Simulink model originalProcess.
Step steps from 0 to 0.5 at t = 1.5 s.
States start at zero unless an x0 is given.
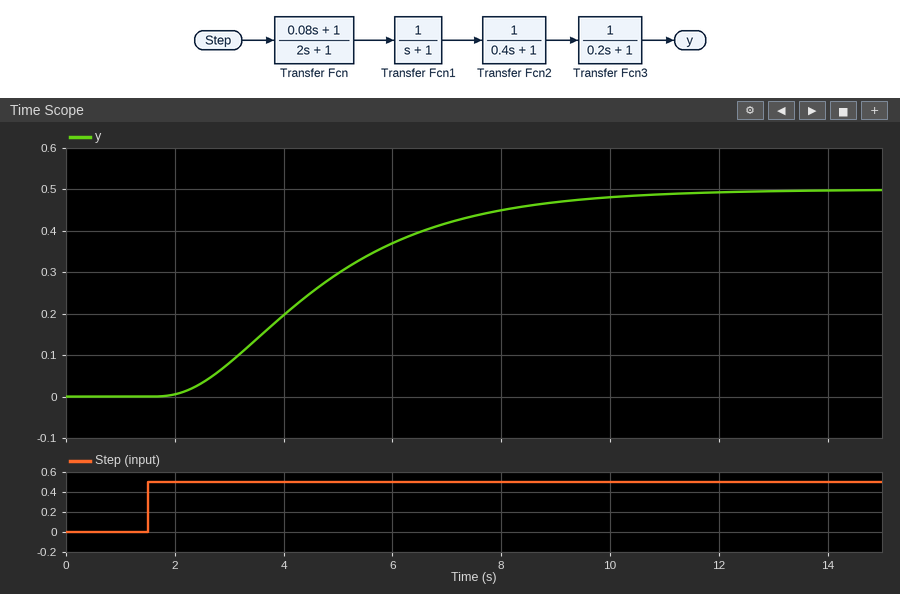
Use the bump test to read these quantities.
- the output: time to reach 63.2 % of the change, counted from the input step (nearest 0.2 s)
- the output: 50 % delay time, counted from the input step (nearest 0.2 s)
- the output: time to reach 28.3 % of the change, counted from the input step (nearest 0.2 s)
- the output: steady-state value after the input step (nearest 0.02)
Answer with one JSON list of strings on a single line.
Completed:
["3.8 s", "3.0 s", "2.0 s", "0.50"]
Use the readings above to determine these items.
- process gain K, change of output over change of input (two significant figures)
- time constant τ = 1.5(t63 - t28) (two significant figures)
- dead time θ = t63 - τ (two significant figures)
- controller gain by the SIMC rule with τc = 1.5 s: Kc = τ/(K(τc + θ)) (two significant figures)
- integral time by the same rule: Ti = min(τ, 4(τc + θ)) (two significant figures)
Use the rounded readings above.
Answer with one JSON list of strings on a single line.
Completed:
["1.0", "2.7 s", "1.1 s", "1.0", "2.7 s"]
